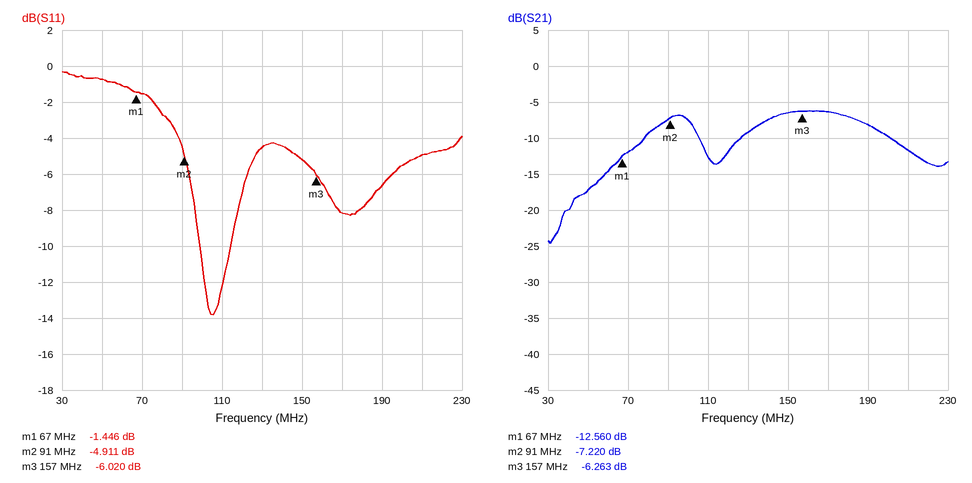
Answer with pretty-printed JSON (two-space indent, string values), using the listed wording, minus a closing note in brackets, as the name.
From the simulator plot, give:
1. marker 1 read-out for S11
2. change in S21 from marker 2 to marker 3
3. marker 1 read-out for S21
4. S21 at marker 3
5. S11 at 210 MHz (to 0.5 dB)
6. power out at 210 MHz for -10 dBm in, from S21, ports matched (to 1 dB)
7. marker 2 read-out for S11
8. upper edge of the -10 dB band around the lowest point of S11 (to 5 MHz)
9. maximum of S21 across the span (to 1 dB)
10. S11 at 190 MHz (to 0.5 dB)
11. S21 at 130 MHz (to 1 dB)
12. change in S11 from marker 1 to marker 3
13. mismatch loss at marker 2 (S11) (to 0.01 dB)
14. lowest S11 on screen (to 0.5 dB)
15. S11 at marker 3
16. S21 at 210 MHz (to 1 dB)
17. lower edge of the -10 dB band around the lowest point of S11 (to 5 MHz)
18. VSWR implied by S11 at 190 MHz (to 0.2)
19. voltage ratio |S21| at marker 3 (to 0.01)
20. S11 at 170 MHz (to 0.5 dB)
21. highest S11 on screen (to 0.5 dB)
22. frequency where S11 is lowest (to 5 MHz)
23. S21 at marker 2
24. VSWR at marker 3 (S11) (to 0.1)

{
  "marker 1 read-out for S11": "-1.446 dB",
  "change in S21 from marker 2 to marker 3": "0.957 dB",
  "marker 1 read-out for S21": "-12.560 dB",
  "S21 at marker 3": "-6.263 dB",
  "S11 at 210 MHz": "-5.0 dB",
  "power out at 210 MHz for -10 dBm in, from S21, ports matched": "-22 dBm",
  "marker 2 read-out for S11": "-4.911 dB",
  "upper edge of the -10 dB band around the lowest point of S11": "115 MHz",
  "maximum of S21 across the span": "-6 dB",
  "S11 at 190 MHz": "-6.5 dB",
  "S21 at 130 MHz": "-9 dB",
  "change in S11 from marker 1 to marker 3": "-4.574 dB",
  "mismatch loss at marker 2 (S11)": "1.69 dB",
  "lowest S11 on screen": "-14.0 dB",
  "S11 at marker 3": "-6.020 dB",
  "S21 at 210 MHz": "-12 dB",
  "lower edge of the -10 dB band around the lowest point of S11": "100 MHz",
  "VSWR implied by S11 at 190 MHz": "2.8",
  "voltage ratio |S21| at marker 3": "0.49",
  "S11 at 170 MHz": "-8.0 dB",
  "highest S11 on screen": "-0.5 dB",
  "frequency where S11 is lowest": "105 MHz",
  "S21 at marker 2": "-7.220 dB",
  "VSWR at marker 3 (S11)": "3.0"
}
